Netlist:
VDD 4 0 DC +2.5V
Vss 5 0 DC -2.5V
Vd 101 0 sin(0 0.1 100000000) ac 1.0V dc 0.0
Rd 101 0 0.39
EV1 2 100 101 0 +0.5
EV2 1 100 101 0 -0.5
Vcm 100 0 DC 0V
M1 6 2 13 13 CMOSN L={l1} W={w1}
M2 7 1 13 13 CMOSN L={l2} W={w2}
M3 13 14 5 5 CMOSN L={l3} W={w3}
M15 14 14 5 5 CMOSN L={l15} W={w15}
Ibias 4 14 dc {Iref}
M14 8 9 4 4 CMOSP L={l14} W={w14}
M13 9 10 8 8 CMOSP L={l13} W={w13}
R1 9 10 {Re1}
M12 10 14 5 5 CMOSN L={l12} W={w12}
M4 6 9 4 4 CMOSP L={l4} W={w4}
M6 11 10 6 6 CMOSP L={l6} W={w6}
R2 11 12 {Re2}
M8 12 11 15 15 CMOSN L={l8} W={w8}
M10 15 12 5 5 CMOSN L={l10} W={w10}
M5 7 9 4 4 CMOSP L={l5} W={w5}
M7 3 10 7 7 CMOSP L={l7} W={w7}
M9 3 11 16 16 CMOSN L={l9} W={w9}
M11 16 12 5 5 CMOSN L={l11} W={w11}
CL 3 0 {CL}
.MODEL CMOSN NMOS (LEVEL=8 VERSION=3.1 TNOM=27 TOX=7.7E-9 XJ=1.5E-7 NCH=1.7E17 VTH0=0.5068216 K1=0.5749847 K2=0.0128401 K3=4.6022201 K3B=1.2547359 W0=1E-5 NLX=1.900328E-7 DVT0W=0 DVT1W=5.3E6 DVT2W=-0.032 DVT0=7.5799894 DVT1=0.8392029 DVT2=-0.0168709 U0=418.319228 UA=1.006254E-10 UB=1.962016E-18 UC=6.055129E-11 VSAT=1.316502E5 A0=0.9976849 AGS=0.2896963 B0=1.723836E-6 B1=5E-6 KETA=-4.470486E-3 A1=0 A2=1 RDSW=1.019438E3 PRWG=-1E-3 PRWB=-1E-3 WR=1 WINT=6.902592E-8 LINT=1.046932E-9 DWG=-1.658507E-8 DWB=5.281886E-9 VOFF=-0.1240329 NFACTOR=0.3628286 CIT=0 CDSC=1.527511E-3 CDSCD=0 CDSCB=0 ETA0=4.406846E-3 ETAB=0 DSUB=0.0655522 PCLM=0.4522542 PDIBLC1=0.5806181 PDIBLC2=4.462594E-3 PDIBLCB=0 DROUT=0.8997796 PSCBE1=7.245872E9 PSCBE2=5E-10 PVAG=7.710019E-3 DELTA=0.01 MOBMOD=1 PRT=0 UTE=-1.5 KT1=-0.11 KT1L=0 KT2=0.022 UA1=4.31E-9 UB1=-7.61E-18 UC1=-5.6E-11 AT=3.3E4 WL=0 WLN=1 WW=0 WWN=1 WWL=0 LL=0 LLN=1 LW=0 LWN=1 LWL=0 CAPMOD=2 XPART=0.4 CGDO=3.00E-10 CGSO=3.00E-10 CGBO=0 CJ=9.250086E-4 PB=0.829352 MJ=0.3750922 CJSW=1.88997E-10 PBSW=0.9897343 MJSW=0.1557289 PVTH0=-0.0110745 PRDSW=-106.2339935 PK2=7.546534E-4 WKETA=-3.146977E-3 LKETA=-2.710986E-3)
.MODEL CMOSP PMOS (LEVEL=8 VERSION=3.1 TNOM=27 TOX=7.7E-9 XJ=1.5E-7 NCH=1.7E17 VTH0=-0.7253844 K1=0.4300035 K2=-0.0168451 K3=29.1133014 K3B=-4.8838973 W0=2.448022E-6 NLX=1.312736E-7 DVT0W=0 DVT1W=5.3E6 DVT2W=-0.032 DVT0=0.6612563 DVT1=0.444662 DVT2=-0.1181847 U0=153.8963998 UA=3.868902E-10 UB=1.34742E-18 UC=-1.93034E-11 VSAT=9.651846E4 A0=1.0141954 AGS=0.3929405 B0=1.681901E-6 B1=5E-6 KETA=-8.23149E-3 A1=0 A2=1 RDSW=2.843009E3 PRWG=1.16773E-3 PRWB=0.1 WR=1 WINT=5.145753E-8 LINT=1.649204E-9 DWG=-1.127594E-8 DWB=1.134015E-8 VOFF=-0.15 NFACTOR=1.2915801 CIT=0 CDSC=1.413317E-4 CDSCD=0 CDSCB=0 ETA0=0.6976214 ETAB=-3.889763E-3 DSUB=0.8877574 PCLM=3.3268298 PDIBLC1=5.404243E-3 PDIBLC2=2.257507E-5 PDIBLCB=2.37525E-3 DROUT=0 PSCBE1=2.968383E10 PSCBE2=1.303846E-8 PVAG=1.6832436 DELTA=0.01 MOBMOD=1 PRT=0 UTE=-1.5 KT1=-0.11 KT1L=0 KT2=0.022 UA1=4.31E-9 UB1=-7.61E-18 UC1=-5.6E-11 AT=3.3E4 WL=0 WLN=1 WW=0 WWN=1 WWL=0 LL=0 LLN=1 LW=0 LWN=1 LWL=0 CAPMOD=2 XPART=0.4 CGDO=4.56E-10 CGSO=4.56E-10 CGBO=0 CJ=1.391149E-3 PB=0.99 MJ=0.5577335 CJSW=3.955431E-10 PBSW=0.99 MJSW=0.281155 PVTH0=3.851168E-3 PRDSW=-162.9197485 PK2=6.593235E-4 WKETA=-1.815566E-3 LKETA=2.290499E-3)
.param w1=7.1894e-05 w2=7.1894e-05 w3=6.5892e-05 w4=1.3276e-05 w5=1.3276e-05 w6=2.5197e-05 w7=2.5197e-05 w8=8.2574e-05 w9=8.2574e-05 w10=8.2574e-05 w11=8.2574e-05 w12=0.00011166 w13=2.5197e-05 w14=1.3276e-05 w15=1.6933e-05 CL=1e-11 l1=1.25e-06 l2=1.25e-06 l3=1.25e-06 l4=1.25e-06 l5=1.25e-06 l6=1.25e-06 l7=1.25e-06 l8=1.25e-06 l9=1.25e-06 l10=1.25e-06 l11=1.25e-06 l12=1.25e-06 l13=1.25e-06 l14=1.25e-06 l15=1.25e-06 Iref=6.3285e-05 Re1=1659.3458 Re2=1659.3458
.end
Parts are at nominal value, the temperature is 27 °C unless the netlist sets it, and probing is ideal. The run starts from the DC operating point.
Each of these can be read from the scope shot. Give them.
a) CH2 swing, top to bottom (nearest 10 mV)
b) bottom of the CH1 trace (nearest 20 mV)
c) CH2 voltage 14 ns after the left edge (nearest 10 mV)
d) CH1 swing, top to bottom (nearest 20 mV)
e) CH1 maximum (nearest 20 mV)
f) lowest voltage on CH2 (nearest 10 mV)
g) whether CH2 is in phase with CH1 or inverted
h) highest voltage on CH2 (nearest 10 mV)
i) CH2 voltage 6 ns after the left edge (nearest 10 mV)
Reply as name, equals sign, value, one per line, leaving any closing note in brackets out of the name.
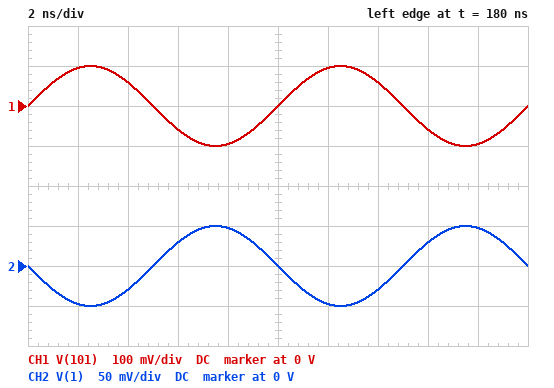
CH2 swing, top to bottom = 100 mV
bottom of the CH1 trace = -100 mV
CH2 voltage 14 ns after the left edge = -30 mV
CH1 swing, top to bottom = 200 mV
CH1 maximum = 100 mV
lowest voltage on CH2 = -50 mV
whether CH2 is in phase with CH1 or inverted = inverted
highest voltage on CH2 = 50 mV
CH2 voltage 6 ns after the left edge = 30 mV
